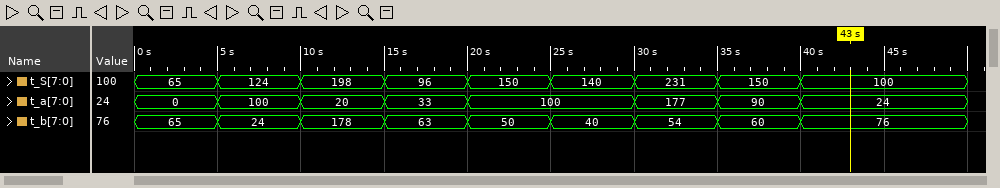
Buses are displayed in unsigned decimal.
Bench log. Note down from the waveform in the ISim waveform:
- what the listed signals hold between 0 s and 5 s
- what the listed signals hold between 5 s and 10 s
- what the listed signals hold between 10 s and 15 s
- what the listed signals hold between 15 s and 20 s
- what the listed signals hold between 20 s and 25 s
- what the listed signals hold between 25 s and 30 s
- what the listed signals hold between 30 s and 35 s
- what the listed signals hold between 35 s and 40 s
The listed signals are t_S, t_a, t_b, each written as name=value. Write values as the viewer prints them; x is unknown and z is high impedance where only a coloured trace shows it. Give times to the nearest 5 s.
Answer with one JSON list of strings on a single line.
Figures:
["t_S=65, t_a=0, t_b=65", "t_S=124, t_a=100, t_b=24", "t_S=198, t_a=20, t_b=178", "t_S=96, t_a=33, t_b=63", "t_S=150, t_a=100, t_b=50", "t_S=140, t_a=100, t_b=40", "t_S=231, t_a=177, t_b=54", "t_S=150, t_a=90, t_b=60"]
